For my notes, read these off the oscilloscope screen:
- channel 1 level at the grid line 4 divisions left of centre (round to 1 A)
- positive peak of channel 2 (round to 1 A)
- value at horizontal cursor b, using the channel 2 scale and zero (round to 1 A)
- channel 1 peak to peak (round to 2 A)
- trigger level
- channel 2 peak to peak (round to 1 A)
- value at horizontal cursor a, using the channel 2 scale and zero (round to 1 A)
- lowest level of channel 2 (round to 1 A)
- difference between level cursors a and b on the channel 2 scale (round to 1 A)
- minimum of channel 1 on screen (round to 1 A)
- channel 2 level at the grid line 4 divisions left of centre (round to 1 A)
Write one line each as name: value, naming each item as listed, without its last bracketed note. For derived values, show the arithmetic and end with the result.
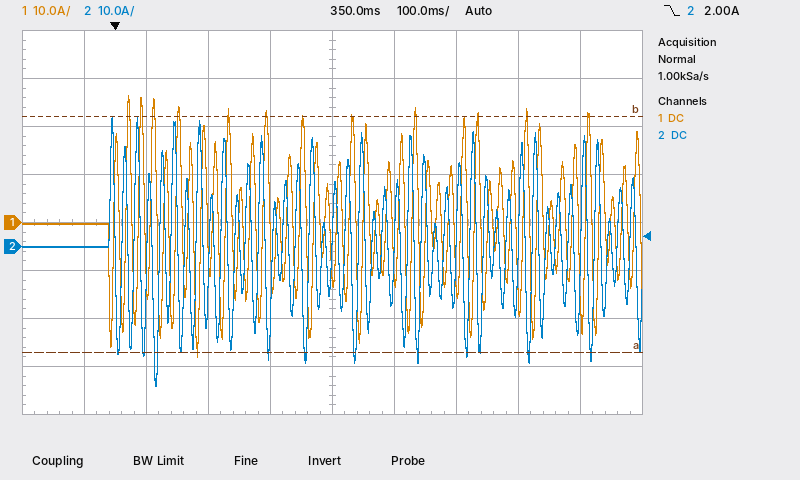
channel 1 level at the grid line 4 divisions left of centre: 0 A
positive peak of channel 2: 27 A
value at horizontal cursor b, using the channel 2 scale and zero: 27 A
channel 1 peak to peak: 54 A
trigger level: 2.00 A
channel 2 peak to peak: 27 A − (-29 A) = 56 A
value at horizontal cursor a, using the channel 2 scale and zero: -22 A
lowest level of channel 2: -29 A
difference between level cursors a and b on the channel 2 scale: 49 A
minimum of channel 1 on screen: -28 A
channel 2 level at the grid line 4 divisions left of centre: 0 A
